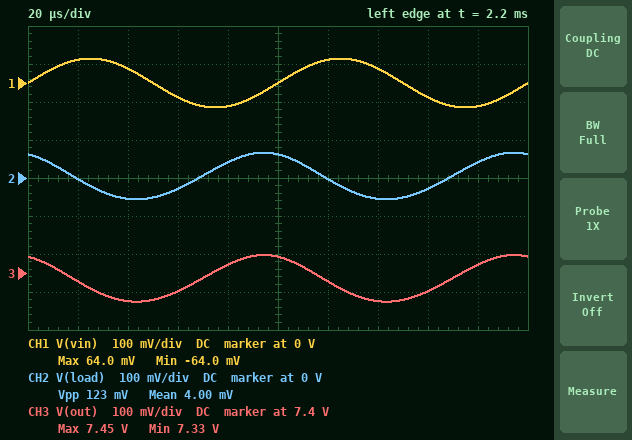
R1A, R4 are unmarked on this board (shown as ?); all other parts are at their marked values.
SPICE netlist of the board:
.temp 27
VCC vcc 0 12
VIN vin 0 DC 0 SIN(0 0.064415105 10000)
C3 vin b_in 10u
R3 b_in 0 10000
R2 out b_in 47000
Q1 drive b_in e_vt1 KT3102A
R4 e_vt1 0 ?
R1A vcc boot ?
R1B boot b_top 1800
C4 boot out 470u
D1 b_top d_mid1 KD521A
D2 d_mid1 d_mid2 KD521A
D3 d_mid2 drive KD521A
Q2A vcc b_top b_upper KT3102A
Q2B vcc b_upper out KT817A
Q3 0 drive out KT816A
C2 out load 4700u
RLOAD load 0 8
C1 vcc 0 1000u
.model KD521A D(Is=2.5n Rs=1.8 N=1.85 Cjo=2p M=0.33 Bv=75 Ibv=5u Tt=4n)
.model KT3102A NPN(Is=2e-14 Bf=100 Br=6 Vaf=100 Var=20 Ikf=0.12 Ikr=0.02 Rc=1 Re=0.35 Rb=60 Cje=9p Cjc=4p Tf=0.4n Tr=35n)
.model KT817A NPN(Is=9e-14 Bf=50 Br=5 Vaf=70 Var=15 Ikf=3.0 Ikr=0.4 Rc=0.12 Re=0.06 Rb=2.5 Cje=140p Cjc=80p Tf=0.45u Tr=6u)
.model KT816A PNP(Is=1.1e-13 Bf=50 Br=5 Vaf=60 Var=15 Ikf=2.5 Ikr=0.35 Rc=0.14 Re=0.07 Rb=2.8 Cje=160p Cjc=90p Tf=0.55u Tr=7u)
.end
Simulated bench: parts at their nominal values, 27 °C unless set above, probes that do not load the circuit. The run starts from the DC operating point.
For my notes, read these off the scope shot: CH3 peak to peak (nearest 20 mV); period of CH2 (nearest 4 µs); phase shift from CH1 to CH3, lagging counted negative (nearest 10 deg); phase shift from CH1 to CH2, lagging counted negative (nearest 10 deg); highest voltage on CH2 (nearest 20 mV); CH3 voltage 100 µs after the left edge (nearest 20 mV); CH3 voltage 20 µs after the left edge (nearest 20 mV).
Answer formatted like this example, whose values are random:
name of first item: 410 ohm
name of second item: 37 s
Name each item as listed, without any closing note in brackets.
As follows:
CH3 peak to peak: 120 mV
period of CH2: 100 µs
phase shift from CH1 to CH3, lagging counted negative: 110 deg
phase shift from CH1 to CH2, lagging counted negative: 110 deg
highest voltage on CH2: 60 mV
CH3 voltage 100 µs after the left edge: 7.44 V
CH3 voltage 20 µs after the left edge: 7.38 V
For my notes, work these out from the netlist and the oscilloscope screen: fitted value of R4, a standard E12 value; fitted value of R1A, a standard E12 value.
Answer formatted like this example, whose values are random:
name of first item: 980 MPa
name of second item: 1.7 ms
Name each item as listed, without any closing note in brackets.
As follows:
fitted value of R4, a standard E12 value: 270 Ω
fitted value of R1A, a standard E12 value: 330 Ω
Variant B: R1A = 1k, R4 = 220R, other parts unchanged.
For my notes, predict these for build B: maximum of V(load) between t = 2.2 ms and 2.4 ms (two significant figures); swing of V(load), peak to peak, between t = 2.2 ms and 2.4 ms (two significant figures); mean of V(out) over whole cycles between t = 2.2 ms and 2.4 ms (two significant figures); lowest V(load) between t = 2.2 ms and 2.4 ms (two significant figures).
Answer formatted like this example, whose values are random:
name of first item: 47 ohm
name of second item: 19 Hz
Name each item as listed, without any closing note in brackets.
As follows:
maximum of V(load) between t = 2.2 ms and 2.4 ms: 87 mV
swing of V(load), peak to peak, between t = 2.2 ms and 2.4 ms: 150 mV
mean of V(out) over whole cycles between t = 2.2 ms and 2.4 ms: 6.6 V
lowest V(load) between t = 2.2 ms and 2.4 ms: -67 mV
